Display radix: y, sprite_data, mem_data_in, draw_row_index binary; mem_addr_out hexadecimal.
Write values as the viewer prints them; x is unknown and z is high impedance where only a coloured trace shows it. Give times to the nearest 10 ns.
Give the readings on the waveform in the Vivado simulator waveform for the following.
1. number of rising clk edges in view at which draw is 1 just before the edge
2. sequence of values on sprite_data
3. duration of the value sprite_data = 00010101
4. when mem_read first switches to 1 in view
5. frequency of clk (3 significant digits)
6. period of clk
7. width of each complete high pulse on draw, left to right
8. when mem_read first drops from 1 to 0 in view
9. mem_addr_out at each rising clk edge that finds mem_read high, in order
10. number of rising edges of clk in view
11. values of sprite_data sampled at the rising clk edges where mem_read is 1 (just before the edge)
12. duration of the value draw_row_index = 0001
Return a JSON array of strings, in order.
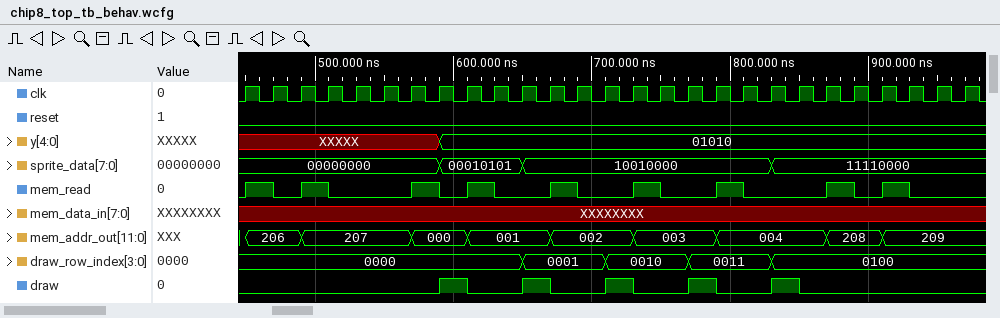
["5", "00000000, 00010101, 10010000, 11110000", "60 ns", "450 ns", "50.0 MHz", "20 ns", "20 ns, 20 ns, 20 ns, 20 ns, 20 ns", "470 ns", "206, 207, 000, 001, 002, 003, 004, 208, 209", "27", "00000000, 00000000, 00000000, 00010101, 10010000, 10010000, 10010000, 11110000, 11110000", "60 ns"]
